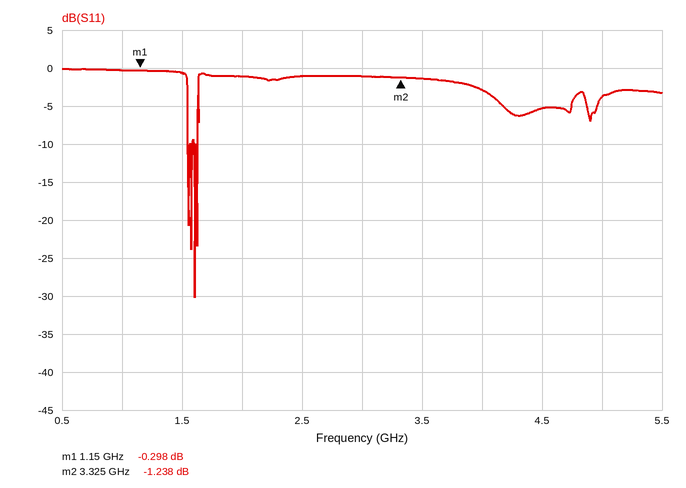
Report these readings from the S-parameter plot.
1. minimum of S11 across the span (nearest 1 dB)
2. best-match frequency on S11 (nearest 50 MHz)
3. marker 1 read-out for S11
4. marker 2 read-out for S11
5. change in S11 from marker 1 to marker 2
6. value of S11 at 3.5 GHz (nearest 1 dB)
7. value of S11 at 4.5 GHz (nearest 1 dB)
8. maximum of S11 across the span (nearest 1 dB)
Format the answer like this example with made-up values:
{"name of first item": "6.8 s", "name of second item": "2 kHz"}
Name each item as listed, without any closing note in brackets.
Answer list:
{"minimum of S11 across the span": "-30 dB", "best-match frequency on S11": "1.60 GHz", "marker 1 read-out for S11": "-0.298 dB", "marker 2 read-out for S11": "-1.238 dB", "change in S11 from marker 1 to marker 2": "-0.940 dB", "value of S11 at 3.5 GHz": "-1 dB", "value of S11 at 4.5 GHz": "-5 dB", "maximum of S11 across the span": "0 dB"}
